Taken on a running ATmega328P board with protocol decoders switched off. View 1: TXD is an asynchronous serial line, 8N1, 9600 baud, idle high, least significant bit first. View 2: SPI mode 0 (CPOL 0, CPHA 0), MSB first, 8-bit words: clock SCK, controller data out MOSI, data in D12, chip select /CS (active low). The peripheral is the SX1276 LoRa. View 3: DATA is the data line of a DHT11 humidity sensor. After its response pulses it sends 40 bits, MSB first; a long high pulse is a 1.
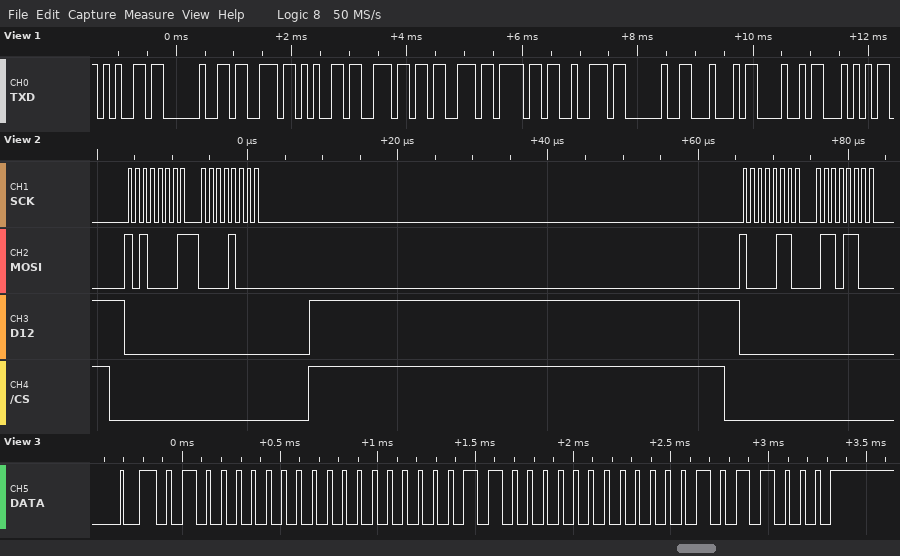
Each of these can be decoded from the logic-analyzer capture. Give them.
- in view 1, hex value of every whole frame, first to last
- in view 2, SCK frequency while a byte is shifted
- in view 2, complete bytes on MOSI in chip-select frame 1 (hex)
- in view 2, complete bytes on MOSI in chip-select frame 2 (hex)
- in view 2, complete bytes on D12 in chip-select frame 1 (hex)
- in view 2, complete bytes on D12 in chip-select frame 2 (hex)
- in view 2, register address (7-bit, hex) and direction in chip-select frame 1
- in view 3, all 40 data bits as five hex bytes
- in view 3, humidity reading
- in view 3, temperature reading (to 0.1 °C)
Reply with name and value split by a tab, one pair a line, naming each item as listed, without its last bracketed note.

in view 1, hex value of every whole frame, first to last	65 20 73 65 6E 73 6F 72 20 44 48 54
in view 2, SCK frequency while a byte is shifted	1 MHz
in view 2, complete bytes on MOSI in chip-select frame 1	A1 08
in view 2, complete bytes on MOSI in chip-select frame 2	86 6C
in view 2, complete bytes on D12 in chip-select frame 1	00 00
in view 2, complete bytes on D12 in chip-select frame 2	00 00
in view 2, register address (7-bit, hex) and direction in chip-select frame 1	0x21 write
in view 3, all 40 data bits as five hex bytes	40 00 18 00 58
in view 3, humidity reading	64 %
in view 3, temperature reading	24.0 °C
